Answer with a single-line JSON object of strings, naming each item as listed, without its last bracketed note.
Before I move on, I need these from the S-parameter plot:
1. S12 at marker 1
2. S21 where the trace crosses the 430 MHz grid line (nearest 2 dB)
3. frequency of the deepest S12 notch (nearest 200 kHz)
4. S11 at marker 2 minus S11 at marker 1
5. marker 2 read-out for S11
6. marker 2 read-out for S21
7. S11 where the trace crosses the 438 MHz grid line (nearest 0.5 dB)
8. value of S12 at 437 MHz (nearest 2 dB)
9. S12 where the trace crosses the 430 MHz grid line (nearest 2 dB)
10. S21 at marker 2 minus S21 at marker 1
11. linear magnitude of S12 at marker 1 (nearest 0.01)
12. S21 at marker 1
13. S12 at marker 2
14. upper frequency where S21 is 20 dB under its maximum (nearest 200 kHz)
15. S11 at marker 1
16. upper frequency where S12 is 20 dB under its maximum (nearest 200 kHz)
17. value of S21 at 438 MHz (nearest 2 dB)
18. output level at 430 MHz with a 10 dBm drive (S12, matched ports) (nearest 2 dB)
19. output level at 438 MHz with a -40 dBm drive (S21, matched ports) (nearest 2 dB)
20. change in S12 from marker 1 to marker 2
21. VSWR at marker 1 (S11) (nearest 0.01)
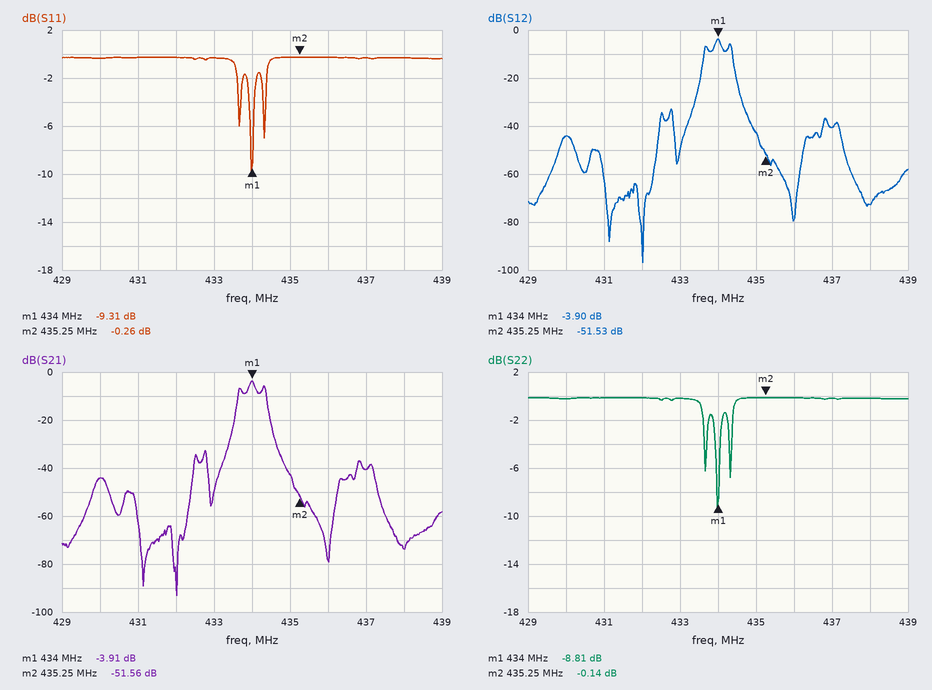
{"S12 at marker 1": "-3.90 dB", "S21 where the trace crosses the 430 MHz grid line": "-44 dB", "frequency of the deepest S12 notch": "432.0 MHz", "S11 at marker 2 minus S11 at marker 1": "9.05 dB", "marker 2 read-out for S11": "-0.26 dB", "marker 2 read-out for S21": "-51.56 dB", "S11 where the trace crosses the 438 MHz grid line": "-0.5 dB", "value of S12 at 437 MHz": "-40 dB", "S12 where the trace crosses the 430 MHz grid line": "-44 dB", "S21 at marker 2 minus S21 at marker 1": "-47.65 dB", "linear magnitude of S12 at marker 1": "0.64", "S21 at marker 1": "-3.91 dB", "S12 at marker 2": "-51.53 dB", "upper frequency where S21 is 20 dB under its maximum": "434.6 MHz", "S11 at marker 1": "-9.31 dB", "upper frequency where S12 is 20 dB under its maximum": "434.6 MHz", "value of S21 at 438 MHz": "-74 dB", "output level at 430 MHz with a 10 dBm drive (S12, matched ports)": "-34 dBm", "output level at 438 MHz with a -40 dBm drive (S21, matched ports)": "-114 dBm", "change in S12 from marker 1 to marker 2": "-47.63 dB", "VSWR at marker 1 (S11)": "2.04"}
